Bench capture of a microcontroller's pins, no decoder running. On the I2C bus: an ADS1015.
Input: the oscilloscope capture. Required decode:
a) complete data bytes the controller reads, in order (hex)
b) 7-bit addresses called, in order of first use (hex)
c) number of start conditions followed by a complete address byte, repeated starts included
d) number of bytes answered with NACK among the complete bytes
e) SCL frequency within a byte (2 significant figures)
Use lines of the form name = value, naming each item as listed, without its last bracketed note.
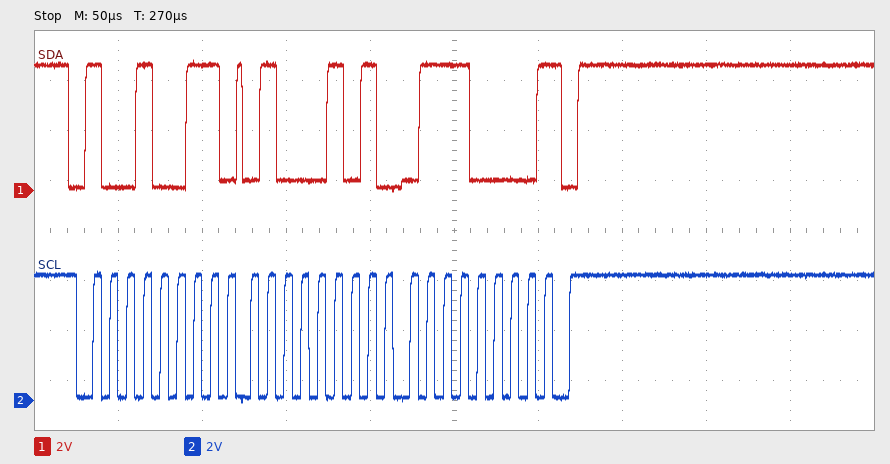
complete data bytes the controller reads, in order = 45 70
7-bit addresses called, in order of first use = 0x49
number of start conditions followed by a complete address byte, repeated starts included = 1
number of bytes answered with NACK among the complete bytes = 1
SCL frequency within a byte = 100 kHz
